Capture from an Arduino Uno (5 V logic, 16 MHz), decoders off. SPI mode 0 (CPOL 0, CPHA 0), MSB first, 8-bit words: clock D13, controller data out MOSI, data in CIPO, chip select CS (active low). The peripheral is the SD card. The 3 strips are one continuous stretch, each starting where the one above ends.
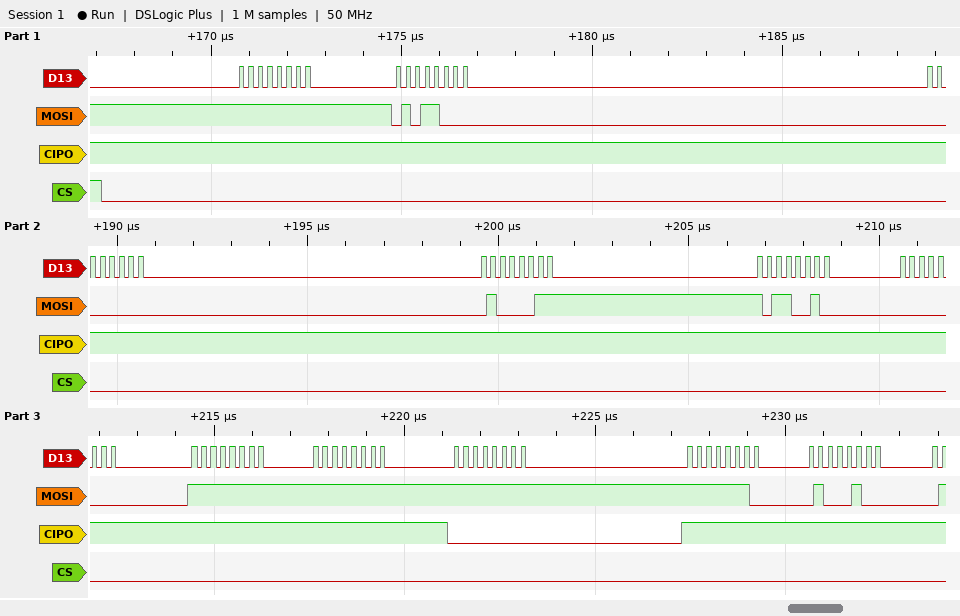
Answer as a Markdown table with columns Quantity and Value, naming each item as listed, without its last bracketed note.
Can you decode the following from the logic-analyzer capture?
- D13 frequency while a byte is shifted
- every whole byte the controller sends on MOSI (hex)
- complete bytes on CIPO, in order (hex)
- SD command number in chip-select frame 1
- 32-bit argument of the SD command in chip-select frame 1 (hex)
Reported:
| Quantity | Value |
|---|---|
| D13 frequency while a byte is shifted | 4 MHz |
| every whole byte the controller sends on MOSI | 0xFF 0x58 0x00 0x43 0xB2 0x00 0xFF 0xFF 0xFF 0xFE 0x44 |
| complete bytes on CIPO, in order | 0xFF 0xFF 0xFF 0xFF 0xFF 0xFF 0xFF 0xFF 0x00 0xFF 0xFF |
| SD command number in chip-select frame 1 | CMD24 |
| 32-bit argument of the SD command in chip-select frame 1 | 0x0043B200 |
